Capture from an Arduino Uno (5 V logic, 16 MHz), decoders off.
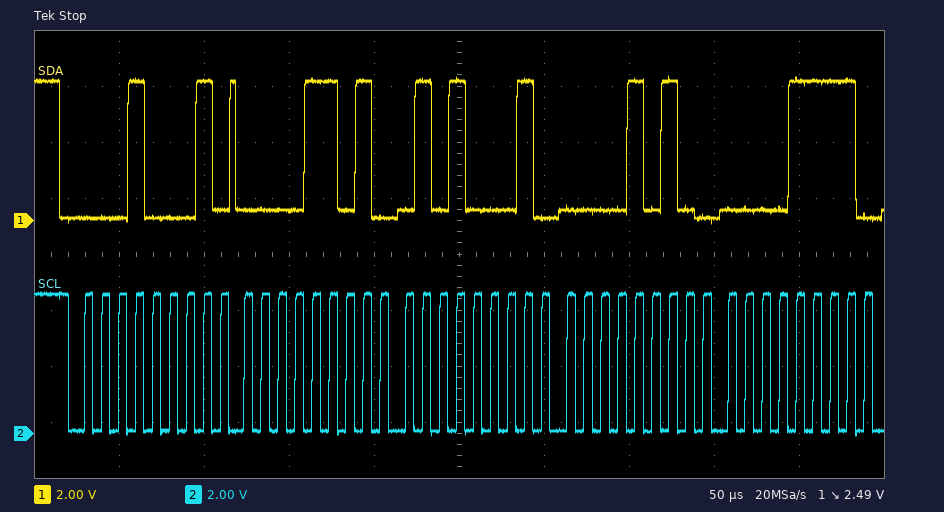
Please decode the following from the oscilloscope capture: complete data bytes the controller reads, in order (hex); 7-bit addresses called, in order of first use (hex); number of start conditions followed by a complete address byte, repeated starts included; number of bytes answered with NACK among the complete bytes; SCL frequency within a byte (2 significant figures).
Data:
0D 51 0A 0F
0x08
1
0
100 kHz
